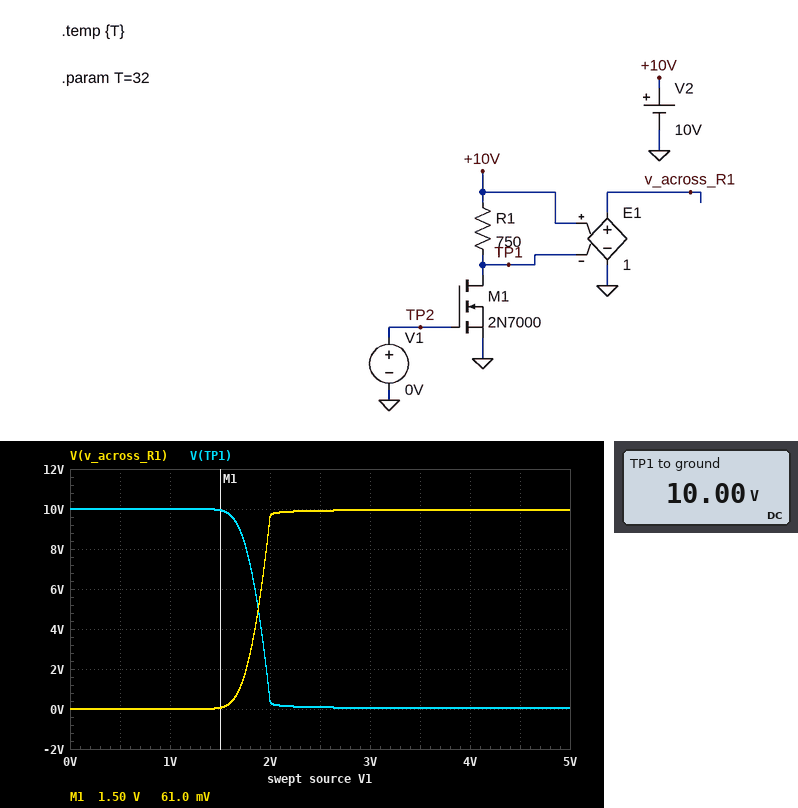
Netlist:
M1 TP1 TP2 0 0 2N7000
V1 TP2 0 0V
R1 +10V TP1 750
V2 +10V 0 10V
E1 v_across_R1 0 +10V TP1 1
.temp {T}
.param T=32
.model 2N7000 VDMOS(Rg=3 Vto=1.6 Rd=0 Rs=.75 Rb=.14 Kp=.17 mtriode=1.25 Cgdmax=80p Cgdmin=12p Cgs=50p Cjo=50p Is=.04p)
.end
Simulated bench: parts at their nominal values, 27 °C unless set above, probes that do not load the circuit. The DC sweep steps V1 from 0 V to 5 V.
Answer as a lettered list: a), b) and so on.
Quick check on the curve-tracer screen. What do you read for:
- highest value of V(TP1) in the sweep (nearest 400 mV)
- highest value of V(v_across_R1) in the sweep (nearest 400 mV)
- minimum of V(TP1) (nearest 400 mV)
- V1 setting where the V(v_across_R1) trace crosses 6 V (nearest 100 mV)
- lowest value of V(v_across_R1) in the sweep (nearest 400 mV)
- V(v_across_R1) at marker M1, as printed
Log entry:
a) 10.0 V
b) 10.0 V
c) 0 V
d) 1.9 V
e) 0 V
f) 61.0 mV
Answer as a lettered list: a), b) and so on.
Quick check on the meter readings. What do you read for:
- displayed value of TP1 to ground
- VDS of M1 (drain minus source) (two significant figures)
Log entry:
a) 10.00 V
b) 10 V
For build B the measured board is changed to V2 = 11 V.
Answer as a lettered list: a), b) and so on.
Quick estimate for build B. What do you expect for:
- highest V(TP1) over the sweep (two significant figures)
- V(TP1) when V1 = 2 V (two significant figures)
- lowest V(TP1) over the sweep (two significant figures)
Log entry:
a) 11 V
b) 1.4 V
c) 32 mV
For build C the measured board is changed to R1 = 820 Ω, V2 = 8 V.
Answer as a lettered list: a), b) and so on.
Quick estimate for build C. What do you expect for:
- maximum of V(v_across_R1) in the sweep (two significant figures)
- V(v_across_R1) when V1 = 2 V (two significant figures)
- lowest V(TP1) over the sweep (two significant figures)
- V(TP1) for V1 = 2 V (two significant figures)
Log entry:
a) 8.0 V
b) 7.8 V
c) 21 mV
d) 160 mV
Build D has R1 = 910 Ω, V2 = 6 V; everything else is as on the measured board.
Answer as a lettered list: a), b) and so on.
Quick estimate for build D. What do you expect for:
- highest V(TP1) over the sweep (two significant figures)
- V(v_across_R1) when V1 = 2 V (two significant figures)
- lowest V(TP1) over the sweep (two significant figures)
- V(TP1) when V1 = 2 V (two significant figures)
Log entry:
a) 6.0 V
b) 5.9 V
c) 14 mV
d) 97 mV
